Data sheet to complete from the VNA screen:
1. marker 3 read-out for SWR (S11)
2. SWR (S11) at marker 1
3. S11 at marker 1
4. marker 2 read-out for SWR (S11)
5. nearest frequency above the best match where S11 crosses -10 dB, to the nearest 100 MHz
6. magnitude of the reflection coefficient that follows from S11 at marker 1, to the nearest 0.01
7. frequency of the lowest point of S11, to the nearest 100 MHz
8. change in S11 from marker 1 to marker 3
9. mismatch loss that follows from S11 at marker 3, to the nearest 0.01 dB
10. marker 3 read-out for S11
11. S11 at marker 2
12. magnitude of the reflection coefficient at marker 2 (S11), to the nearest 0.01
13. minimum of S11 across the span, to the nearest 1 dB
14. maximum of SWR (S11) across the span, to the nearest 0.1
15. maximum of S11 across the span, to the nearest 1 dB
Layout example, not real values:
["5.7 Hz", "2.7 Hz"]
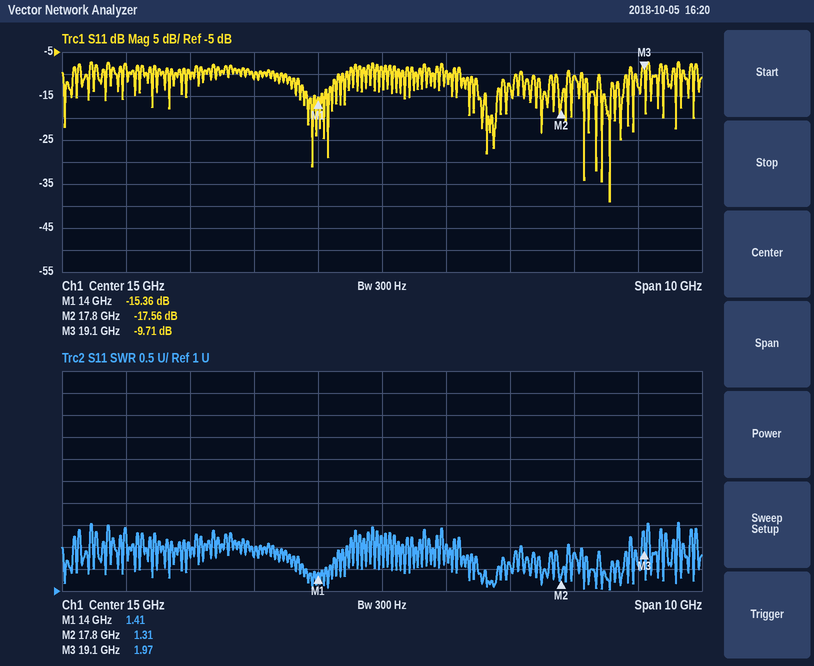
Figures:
["1.97", "1.41", "-15.36 dB", "1.31", "18.9 GHz", "0.17", "18.6 GHz", "5.65 dB", "0.49 dB", "-9.71 dB", "-17.56 dB", "0.13", "-39 dB", "2.6", "-7 dB"]
